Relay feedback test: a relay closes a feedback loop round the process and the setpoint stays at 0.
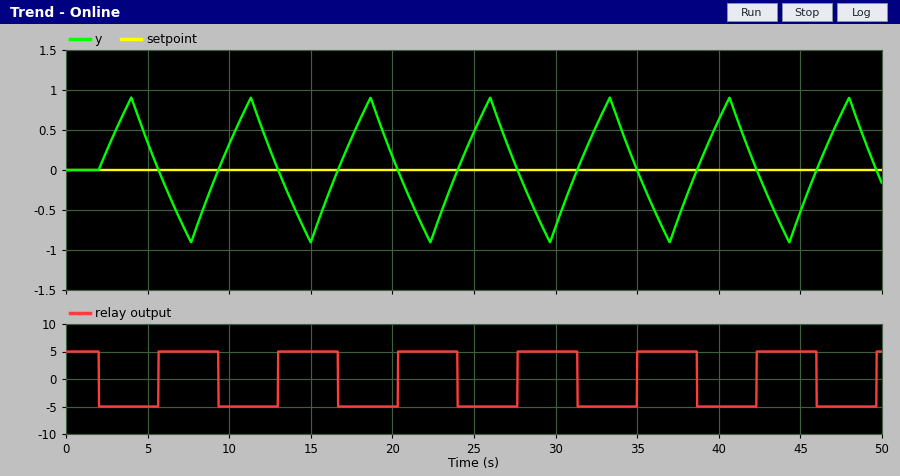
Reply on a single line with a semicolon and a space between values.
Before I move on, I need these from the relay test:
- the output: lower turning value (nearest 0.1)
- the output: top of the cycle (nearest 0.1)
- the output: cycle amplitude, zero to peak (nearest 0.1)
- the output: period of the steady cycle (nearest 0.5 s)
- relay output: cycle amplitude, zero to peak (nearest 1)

-0.9; 0.9; 0.9; 7.5 s; 5
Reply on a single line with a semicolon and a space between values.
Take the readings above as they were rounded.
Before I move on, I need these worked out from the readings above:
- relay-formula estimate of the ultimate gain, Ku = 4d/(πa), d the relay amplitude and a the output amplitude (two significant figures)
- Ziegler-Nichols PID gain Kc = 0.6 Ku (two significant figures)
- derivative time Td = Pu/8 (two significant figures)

7.1; 4.3; 0.94 s
